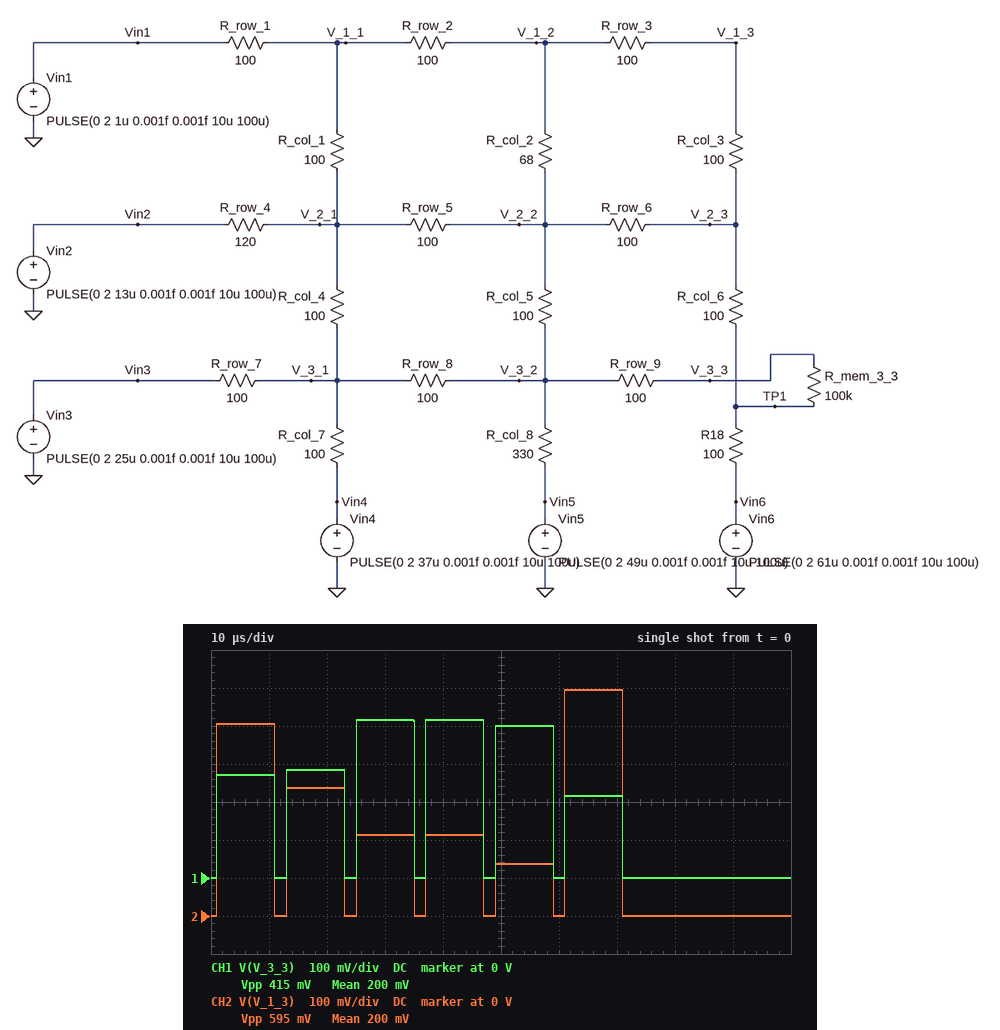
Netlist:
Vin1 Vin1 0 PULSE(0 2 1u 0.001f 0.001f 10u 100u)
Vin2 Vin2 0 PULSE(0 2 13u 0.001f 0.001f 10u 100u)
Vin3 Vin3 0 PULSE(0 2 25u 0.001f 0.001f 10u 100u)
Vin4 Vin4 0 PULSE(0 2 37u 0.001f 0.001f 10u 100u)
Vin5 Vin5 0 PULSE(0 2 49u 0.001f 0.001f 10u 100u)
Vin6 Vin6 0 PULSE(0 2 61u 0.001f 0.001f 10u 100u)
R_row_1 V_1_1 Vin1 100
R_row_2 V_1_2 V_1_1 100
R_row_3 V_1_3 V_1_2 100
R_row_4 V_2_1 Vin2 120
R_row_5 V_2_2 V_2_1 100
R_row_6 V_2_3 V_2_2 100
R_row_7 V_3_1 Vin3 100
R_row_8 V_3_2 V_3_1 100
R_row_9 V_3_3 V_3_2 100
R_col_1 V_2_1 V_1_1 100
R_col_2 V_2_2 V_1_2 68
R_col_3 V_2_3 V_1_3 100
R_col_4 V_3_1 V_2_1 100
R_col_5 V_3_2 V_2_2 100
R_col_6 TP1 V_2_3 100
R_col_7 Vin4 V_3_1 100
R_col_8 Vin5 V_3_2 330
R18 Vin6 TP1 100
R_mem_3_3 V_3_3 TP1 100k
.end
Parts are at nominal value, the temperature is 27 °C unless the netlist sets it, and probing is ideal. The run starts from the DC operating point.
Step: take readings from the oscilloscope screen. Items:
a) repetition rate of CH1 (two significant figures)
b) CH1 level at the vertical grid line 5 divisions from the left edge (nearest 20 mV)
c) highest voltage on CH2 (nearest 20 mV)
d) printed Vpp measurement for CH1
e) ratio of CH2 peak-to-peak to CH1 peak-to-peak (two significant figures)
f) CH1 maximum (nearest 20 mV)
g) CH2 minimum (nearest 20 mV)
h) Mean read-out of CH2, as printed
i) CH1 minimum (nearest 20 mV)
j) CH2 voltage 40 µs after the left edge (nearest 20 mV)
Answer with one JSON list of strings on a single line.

["83 kHz", "400 mV", "600 mV", "415 mV", "1.4", "420 mV", "0 V", "200 mV", "0 V", "220 mV"]
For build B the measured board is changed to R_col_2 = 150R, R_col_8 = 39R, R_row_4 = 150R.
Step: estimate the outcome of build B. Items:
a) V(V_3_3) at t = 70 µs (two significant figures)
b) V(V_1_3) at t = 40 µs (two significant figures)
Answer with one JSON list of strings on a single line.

["89 mV", "130 mV"]
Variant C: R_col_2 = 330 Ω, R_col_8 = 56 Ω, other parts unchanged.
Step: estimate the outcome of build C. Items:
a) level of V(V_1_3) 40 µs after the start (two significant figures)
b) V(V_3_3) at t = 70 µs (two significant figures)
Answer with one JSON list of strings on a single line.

["130 mV", "110 mV"]
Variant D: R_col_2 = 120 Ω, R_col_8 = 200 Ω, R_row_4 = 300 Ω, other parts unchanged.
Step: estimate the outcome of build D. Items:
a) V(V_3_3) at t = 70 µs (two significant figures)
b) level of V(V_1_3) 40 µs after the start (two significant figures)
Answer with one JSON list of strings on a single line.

["210 mV", "230 mV"]
